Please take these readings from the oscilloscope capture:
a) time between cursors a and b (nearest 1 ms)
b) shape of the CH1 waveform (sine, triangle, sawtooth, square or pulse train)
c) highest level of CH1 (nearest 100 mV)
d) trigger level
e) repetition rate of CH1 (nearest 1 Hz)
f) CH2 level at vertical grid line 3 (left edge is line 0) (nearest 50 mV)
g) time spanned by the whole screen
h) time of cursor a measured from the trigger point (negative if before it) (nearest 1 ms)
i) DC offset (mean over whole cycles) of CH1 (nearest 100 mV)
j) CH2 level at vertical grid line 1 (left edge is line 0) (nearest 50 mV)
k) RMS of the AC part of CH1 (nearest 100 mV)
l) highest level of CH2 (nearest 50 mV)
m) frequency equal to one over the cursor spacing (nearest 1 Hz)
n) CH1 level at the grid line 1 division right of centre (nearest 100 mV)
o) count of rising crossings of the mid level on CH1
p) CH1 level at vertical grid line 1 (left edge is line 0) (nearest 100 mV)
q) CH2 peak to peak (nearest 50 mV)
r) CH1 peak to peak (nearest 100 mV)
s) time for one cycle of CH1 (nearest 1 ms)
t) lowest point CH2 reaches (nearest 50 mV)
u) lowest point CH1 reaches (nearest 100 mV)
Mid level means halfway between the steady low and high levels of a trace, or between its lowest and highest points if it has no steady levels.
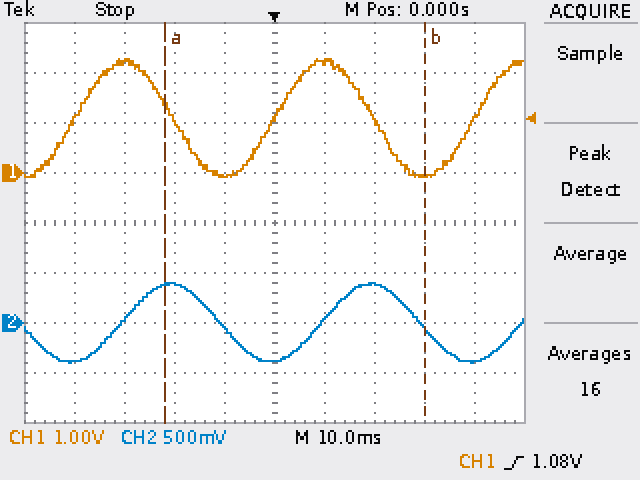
52 ms
sine
2.3 V
1.08 V
25 Hz
400 mV
100 ms
-22 ms
1.1 V
-400 mV
800 mV
400 mV
19 Hz
2.2 V
3
1.1 V
800 mV
2.4 V
40 ms
-400 mV
-100 mV
